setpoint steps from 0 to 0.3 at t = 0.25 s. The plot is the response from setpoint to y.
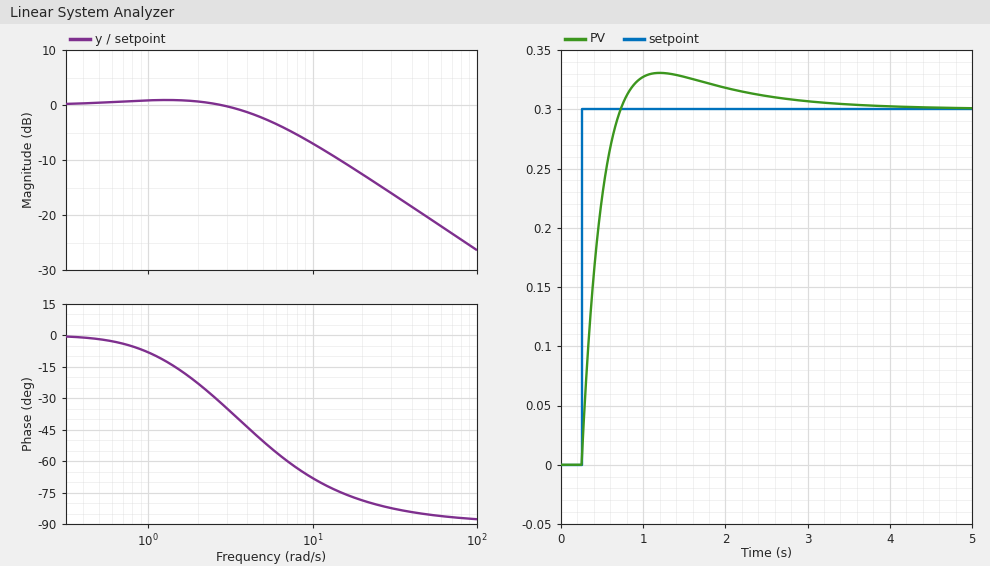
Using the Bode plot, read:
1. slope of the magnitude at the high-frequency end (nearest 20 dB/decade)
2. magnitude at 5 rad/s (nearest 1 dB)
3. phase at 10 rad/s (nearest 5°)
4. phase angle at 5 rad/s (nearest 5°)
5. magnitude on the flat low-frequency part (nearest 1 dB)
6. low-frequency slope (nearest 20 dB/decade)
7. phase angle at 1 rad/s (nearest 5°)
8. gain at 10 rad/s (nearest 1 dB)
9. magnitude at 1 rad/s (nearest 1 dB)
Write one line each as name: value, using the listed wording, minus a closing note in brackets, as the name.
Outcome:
slope of the magnitude at the high-frequency end: -20 dB/decade
magnitude at 5 rad/s: -2 dB
phase at 10 rad/s: -70°
phase angle at 5 rad/s: -50°
magnitude on the flat low-frequency part: 0 dB
low-frequency slope: 0 dB/decade
phase angle at 1 rad/s: -10°
gain at 10 rad/s: -7 dB
magnitude at 1 rad/s: 1 dB
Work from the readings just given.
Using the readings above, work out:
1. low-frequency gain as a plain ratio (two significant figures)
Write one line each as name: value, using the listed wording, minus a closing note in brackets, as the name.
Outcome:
low-frequency gain as a plain ratio: 1.0
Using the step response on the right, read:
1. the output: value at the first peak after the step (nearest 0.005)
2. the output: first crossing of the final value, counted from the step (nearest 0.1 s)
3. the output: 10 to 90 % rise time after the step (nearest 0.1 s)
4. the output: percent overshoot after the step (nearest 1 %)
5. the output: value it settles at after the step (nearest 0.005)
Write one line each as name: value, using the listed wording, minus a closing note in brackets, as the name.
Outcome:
the output: value at the first peak after the step: 0.330
the output: first crossing of the final value, counted from the step: 0.5 s
the output: 10 to 90 % rise time after the step: 0.3 s
the output: percent overshoot after the step: 10 %
the output: value it settles at after the step: 0.300
